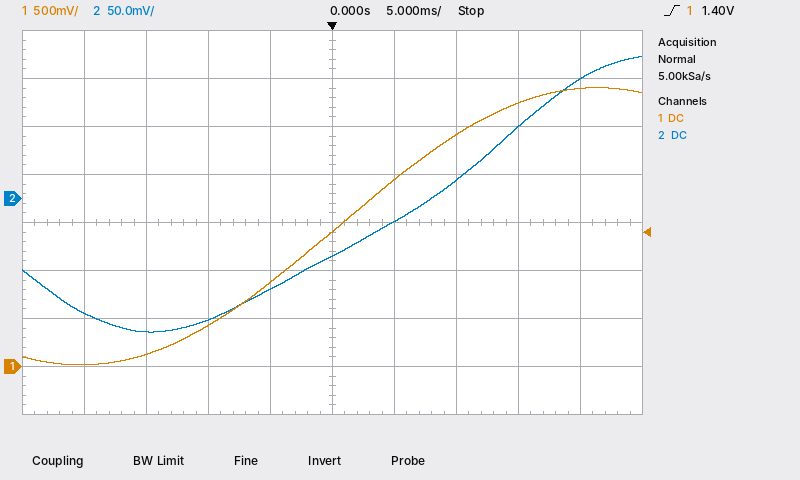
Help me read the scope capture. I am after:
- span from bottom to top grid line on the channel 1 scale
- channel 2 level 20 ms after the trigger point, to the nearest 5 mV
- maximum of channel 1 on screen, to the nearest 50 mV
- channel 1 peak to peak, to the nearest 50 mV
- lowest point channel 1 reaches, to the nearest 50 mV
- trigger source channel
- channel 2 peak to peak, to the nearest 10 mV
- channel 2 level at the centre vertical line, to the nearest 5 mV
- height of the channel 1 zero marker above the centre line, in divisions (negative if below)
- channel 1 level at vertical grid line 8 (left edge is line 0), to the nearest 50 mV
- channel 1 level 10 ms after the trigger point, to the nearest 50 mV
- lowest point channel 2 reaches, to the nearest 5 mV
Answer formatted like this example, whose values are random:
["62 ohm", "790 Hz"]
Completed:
["4 V", "125 mV", "2.90 V", "2.90 V", "0 mV", "channel 1", "290 mV", "-60 mV", "-3.0 div", "2.75 V", "2.40 V", "-140 mV"]
